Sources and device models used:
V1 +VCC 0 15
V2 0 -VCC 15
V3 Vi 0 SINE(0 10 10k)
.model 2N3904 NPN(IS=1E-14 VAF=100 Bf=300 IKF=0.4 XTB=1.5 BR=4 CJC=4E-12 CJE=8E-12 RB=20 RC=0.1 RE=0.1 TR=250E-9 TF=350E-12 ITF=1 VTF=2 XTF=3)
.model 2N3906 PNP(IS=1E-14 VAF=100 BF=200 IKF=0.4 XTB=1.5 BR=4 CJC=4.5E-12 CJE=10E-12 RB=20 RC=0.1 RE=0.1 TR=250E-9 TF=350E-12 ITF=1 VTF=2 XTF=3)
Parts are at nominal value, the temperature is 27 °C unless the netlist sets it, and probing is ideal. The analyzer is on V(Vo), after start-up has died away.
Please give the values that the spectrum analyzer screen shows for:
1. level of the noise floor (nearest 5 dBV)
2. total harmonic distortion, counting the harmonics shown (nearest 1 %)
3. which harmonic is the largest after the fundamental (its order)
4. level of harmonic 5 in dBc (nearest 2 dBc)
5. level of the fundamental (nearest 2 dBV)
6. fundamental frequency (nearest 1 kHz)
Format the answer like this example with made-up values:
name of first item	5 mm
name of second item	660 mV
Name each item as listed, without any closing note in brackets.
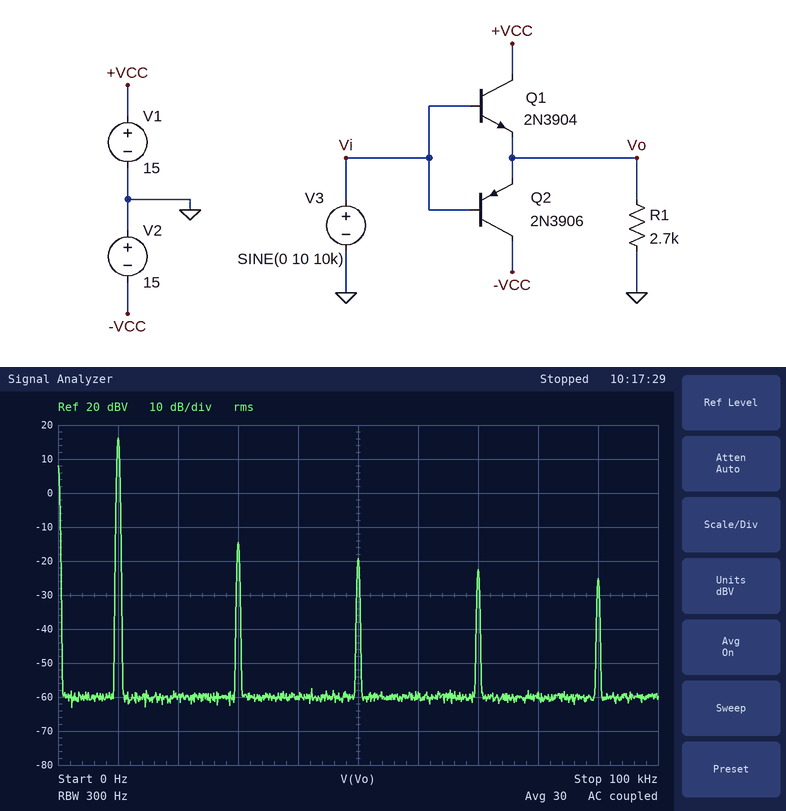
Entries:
level of the noise floor	-60 dBV
total harmonic distortion, counting the harmonics shown	4 %
which harmonic is the largest after the fundamental	3
level of harmonic 5 in dBc	-36 dBc
level of the fundamental	16 dBV
fundamental frequency	10 kHz
